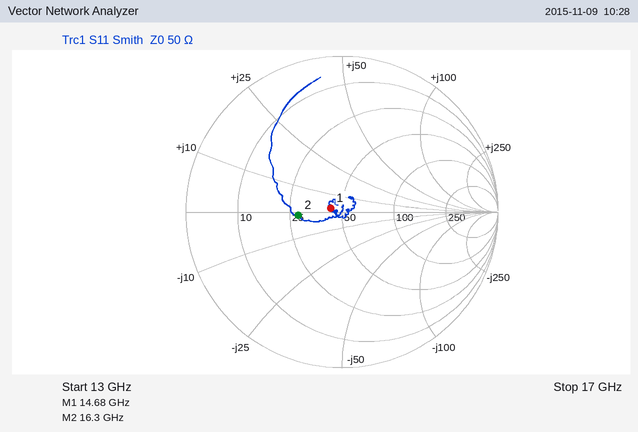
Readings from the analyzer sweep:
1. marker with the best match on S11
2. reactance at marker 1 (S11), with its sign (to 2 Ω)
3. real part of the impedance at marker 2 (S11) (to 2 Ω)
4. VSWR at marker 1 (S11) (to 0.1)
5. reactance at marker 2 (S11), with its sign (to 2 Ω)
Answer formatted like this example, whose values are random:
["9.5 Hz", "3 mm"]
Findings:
["marker 1", "+2 Ω", "28 Ω", "1.2", "-2 Ω"]
